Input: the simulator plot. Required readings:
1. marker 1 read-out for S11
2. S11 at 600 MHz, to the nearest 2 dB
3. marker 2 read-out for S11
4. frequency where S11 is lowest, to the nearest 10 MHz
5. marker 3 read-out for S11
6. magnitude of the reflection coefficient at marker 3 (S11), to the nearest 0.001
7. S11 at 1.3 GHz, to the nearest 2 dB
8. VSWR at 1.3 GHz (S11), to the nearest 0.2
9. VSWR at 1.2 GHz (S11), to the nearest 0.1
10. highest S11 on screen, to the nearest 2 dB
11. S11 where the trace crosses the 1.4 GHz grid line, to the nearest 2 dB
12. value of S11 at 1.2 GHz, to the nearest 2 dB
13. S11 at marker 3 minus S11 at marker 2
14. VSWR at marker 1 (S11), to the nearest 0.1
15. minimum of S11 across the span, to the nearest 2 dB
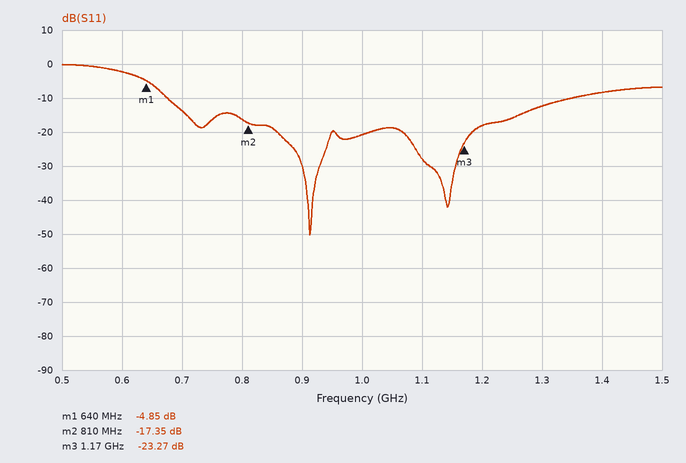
-4.85 dB
-2 dB
-17.35 dB
910 MHz
-23.27 dB
0.069
-12 dB
1.6
1.3
0 dB
-8 dB
-18 dB
-5.92 dB
3.7
-50 dB
